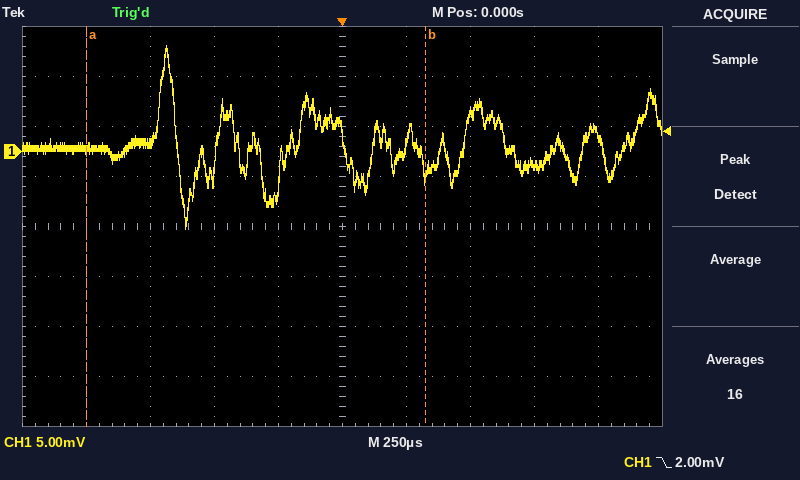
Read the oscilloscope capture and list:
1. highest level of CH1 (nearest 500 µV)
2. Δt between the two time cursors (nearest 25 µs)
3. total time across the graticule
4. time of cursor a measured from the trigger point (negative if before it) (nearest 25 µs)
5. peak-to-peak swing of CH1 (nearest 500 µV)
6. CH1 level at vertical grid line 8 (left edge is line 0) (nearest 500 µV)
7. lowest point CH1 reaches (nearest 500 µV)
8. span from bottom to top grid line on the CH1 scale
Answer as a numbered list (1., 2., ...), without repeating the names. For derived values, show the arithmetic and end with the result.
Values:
1. 10.5 mV
2. 1.325 ms
3. 2.5 ms
4. -1.000 ms
5. 10.5 mV − (-8.0 mV) = 18.5 mV
6. -1.5 mV
7. -8.0 mV
8. 40 mV
